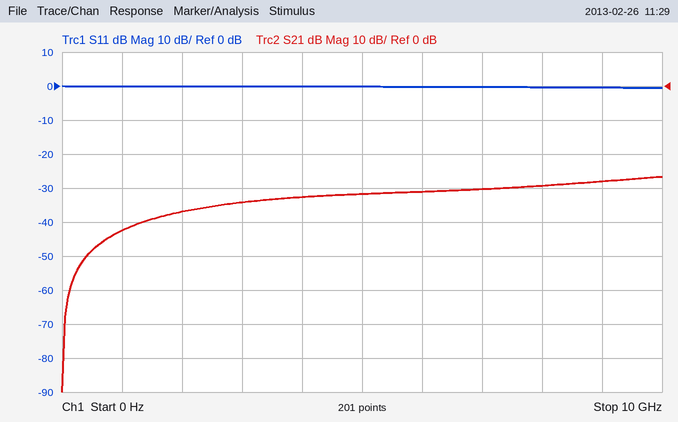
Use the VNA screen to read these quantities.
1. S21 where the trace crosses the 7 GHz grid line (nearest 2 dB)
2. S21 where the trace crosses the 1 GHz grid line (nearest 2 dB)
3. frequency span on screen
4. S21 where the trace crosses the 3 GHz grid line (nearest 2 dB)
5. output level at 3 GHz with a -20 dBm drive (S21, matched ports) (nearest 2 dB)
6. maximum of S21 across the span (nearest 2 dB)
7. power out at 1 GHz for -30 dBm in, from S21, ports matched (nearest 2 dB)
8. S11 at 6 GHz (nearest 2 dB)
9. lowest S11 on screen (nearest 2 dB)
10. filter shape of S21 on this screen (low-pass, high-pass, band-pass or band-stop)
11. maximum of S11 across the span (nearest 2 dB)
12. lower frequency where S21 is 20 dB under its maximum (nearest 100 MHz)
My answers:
-30 dB
-42 dB
10 GHz
-34 dB
-54 dBm
-26 dB
-72 dBm
0 dB
0 dB
high-pass
0 dB
600 MHz
